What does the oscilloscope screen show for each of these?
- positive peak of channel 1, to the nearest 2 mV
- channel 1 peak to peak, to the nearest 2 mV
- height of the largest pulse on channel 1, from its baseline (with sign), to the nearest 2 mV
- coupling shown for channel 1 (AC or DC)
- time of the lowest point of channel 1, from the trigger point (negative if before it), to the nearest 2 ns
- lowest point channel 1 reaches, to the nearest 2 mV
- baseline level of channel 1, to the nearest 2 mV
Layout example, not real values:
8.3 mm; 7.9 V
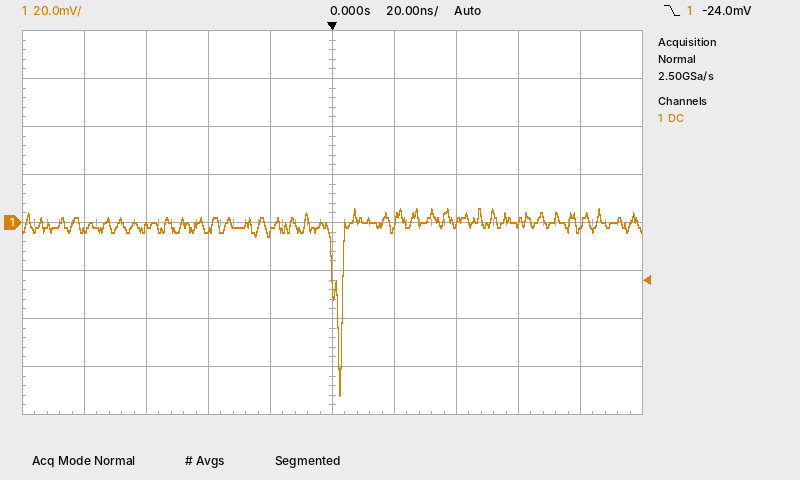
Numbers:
6 mV; 78 mV; -72 mV; DC; +2 ns; -72 mV; 0 mV
